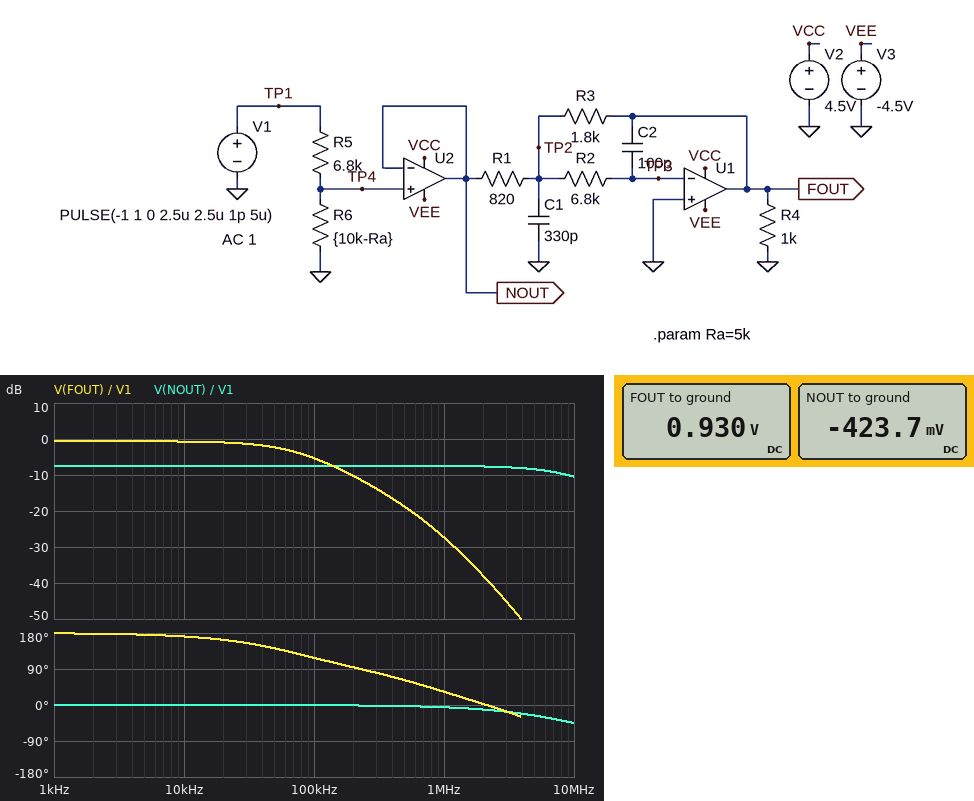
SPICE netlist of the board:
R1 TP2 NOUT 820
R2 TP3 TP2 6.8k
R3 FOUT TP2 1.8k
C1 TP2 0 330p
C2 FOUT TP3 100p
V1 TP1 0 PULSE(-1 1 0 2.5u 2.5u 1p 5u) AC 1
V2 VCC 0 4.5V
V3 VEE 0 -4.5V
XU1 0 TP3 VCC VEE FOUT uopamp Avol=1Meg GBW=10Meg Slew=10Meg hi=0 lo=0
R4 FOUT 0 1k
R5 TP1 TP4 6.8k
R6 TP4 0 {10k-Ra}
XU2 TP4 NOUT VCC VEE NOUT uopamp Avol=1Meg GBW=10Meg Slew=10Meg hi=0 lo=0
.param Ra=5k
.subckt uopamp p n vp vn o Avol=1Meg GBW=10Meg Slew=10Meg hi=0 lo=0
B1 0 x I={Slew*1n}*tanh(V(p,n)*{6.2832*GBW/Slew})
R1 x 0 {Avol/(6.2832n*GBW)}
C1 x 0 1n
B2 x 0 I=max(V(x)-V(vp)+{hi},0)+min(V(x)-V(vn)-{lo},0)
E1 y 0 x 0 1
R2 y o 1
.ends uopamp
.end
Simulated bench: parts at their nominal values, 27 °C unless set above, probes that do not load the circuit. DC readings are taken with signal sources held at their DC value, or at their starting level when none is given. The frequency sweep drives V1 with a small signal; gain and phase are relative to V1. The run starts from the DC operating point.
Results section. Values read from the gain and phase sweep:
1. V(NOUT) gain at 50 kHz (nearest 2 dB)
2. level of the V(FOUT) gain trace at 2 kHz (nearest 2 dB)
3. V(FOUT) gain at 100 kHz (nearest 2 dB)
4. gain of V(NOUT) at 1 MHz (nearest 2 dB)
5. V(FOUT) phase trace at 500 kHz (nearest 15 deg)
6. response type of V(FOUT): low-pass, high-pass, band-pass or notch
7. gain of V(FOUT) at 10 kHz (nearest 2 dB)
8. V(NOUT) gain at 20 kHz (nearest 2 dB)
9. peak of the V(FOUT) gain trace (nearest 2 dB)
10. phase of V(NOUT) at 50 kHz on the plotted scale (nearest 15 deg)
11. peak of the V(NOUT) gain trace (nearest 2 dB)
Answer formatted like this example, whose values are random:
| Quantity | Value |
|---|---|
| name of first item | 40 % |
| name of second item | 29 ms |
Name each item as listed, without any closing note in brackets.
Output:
| Quantity | Value |
|---|---|
| V(NOUT) gain at 50 kHz | -8 dB |
| level of the V(FOUT) gain trace at 2 kHz | 0 dB |
| V(FOUT) gain at 100 kHz | -6 dB |
| gain of V(NOUT) at 1 MHz | -8 dB |
| V(FOUT) phase trace at 500 kHz | 60 deg |
| response type of V(FOUT): low-pass, high-pass, band-pass or notch | low-pass |
| gain of V(FOUT) at 10 kHz | 0 dB |
| V(NOUT) gain at 20 kHz | -8 dB |
| peak of the V(FOUT) gain trace | 0 dB |
| phase of V(NOUT) at 50 kHz on the plotted scale | 0 deg |
| peak of the V(NOUT) gain trace | -8 dB |
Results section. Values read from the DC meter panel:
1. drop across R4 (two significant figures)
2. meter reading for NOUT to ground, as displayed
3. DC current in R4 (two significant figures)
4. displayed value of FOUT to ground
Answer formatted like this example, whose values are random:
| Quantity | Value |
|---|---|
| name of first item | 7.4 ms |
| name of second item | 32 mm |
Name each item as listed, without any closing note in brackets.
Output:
| Quantity | Value |
|---|---|
| drop across R4 | 930 mV |
| meter reading for NOUT to ground, as displayed | -423.7 mV |
| DC current in R4 | 930 µA |
| displayed value of FOUT to ground | 0.930 V |
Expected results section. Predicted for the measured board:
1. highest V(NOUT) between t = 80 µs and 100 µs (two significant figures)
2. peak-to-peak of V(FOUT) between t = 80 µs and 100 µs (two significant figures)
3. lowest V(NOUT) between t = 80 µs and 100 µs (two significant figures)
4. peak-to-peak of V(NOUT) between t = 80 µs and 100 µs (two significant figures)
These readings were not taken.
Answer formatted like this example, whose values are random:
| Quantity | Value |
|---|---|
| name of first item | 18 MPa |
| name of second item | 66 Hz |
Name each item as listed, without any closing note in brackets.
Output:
| Quantity | Value |
|---|---|
| highest V(NOUT) between t = 80 µs and 100 µs | 420 mV |
| peak-to-peak of V(FOUT) between t = 80 µs and 100 µs | 490 mV |
| lowest V(NOUT) between t = 80 µs and 100 µs | -420 mV |
| peak-to-peak of V(NOUT) between t = 80 µs and 100 µs | 840 mV |
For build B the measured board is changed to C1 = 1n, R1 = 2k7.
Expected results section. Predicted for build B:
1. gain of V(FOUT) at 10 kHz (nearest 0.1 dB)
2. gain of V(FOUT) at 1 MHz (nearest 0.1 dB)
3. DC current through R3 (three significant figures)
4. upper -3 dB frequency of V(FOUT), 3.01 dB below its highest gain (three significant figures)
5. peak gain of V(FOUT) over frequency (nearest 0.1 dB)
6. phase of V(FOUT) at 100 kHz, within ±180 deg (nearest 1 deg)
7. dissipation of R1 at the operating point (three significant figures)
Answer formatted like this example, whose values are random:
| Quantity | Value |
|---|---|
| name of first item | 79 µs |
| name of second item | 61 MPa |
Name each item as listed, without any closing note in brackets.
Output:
| Quantity | Value |
|---|---|
| gain of V(FOUT) at 10 kHz | -11.0 dB |
| gain of V(FOUT) at 1 MHz | -44.9 dB |
| DC current through R3 | 157 µA |
| upper -3 dB frequency of V(FOUT), 3.01 dB below its highest gain | 159 kHz |
| peak gain of V(FOUT) over frequency | -10.6 dB |
| phase of V(FOUT) at 100 kHz, within ±180 deg | 120 deg |
| dissipation of R1 at the operating point | 66.5 µW |
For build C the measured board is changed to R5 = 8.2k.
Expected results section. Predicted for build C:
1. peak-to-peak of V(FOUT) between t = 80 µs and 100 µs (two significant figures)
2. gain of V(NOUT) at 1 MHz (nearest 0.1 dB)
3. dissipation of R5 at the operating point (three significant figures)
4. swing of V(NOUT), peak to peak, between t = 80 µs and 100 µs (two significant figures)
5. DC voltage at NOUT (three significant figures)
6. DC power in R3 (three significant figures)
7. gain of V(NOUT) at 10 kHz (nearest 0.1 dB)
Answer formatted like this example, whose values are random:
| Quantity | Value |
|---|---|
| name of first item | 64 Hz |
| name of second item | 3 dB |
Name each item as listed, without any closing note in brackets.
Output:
| Quantity | Value |
|---|---|
| peak-to-peak of V(FOUT) between t = 80 µs and 100 µs | 440 mV |
| gain of V(NOUT) at 1 MHz | -8.5 dB |
| dissipation of R5 at the operating point | 47.1 µW |
| swing of V(NOUT), peak to peak, between t = 80 µs and 100 µs | 750 mV |
| DC voltage at NOUT | -379 mV |
| DC power in R3 | 384 µW |
| gain of V(NOUT) at 10 kHz | -8.4 dB |
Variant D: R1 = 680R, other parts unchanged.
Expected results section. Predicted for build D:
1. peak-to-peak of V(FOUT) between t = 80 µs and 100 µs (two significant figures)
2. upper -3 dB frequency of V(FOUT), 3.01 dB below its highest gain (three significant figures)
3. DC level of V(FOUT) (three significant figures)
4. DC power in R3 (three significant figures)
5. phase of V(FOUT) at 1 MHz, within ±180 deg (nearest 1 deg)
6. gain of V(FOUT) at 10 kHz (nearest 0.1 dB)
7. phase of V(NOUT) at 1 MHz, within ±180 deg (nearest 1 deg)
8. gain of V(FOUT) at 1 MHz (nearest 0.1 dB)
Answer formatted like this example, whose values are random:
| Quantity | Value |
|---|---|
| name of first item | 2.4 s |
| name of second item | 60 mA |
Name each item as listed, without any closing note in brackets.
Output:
| Quantity | Value |
|---|---|
| peak-to-peak of V(FOUT) between t = 80 µs and 100 µs | 520 mV |
| upper -3 dB frequency of V(FOUT), 3.01 dB below its highest gain | 62.4 kHz |
| DC level of V(FOUT) | 1.12 V |
| DC power in R3 | 699 µW |
| phase of V(FOUT) at 1 MHz, within ±180 deg | 37 deg |
| gain of V(FOUT) at 10 kHz | 0.9 dB |
| phase of V(NOUT) at 1 MHz, within ±180 deg | -6 deg |
| gain of V(FOUT) at 1 MHz | -26.3 dB |
